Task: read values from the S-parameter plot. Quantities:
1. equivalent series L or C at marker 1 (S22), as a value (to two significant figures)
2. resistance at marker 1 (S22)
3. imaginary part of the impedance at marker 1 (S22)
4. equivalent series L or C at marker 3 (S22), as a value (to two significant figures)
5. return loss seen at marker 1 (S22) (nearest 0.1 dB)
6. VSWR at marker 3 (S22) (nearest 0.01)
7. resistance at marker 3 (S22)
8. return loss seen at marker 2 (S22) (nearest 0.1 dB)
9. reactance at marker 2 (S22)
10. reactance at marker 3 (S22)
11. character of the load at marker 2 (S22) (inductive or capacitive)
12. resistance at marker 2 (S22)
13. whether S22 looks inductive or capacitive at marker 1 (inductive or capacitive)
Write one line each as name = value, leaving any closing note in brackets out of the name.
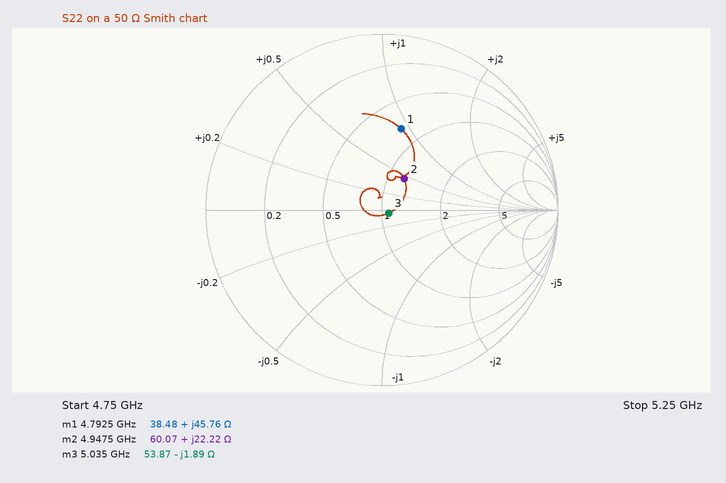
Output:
equivalent series L or C at marker 1 (S22), as a value = 1.5 nH
resistance at marker 1 = 38.48 Ω
imaginary part of the impedance at marker 1 = +45.76 Ω
equivalent series L or C at marker 3 (S22), as a value = 17 pF
return loss seen at marker 1 (S22) = 6.5 dB
VSWR at marker 3 (S22) = 1.09
resistance at marker 3 = 53.87 Ω
return loss seen at marker 2 (S22) = 13.3 dB
reactance at marker 2 = +22.22 Ω
reactance at marker 3 = -1.89 Ω
character of the load at marker 2 (S22) = inductive
resistance at marker 2 = 60.07 Ω
whether S22 looks inductive or capacitive at marker 1 = inductive
